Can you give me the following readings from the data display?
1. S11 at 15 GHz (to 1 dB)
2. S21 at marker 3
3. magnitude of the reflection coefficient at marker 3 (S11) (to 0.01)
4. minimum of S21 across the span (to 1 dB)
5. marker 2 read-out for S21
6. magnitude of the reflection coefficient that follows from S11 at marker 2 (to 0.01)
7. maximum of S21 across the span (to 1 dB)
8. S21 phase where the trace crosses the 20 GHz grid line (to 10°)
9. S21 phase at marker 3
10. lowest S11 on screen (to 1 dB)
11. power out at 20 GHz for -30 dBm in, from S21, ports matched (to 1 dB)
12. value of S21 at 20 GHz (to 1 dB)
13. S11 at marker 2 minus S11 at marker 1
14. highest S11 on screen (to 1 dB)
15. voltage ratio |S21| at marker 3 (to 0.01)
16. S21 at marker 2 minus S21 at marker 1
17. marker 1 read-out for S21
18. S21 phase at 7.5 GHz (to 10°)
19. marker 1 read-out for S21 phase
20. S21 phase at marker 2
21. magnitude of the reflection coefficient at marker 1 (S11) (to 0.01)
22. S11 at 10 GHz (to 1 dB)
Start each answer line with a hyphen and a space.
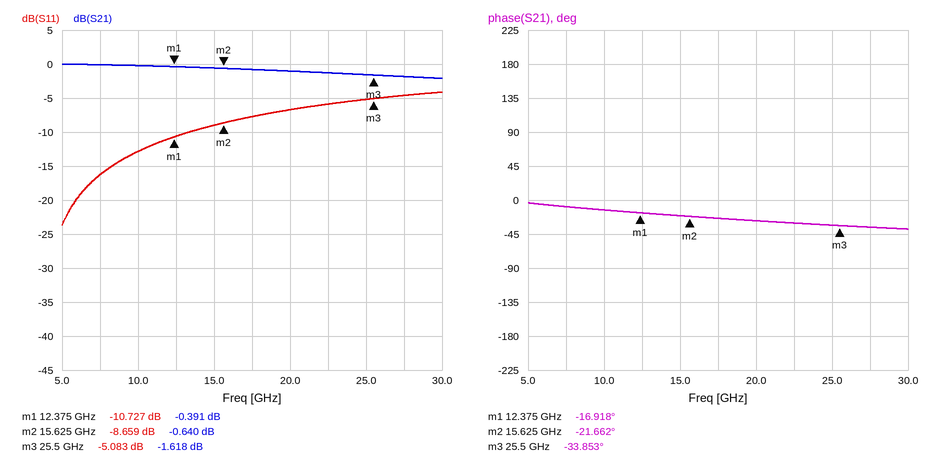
- -9 dB
- -1.618 dB
- 0.56
- -2 dB
- -0.640 dB
- 0.37
- 0 dB
- -30°
- -33.853°
- -24 dB
- -31 dBm
- -1 dB
- 2.068 dB
- -4 dB
- 0.83
- -0.249 dB
- -0.391 dB
- -10°
- -16.918°
- -21.662°
- 0.29
- -13 dB
